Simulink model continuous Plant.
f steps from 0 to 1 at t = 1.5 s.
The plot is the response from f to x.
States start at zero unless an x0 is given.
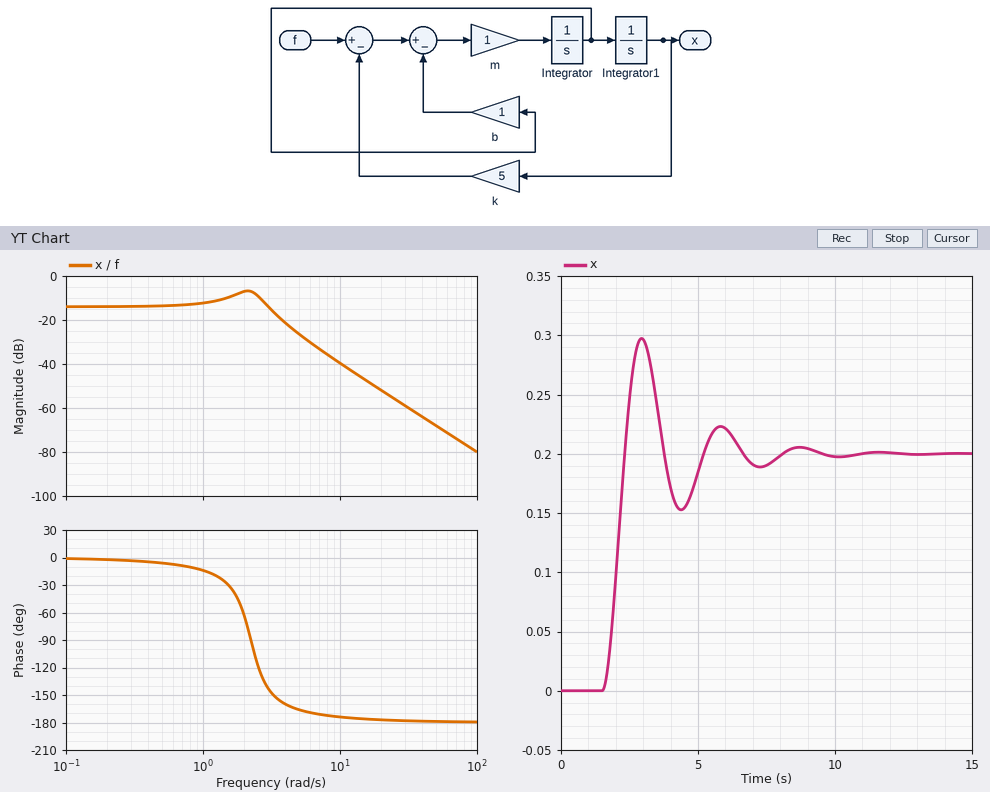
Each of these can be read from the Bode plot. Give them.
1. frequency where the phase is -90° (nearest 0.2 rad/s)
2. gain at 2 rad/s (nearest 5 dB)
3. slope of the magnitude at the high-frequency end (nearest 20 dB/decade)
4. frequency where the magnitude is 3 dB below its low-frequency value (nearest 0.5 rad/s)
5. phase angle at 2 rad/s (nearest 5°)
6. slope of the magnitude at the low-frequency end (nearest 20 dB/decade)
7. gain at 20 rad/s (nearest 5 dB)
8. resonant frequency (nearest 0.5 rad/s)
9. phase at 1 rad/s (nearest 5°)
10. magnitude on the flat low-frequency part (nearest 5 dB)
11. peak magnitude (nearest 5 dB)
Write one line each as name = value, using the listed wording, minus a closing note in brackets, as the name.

frequency where the phase is -90° = 2.2 rad/s
gain at 2 rad/s = -5 dB
slope of the magnitude at the high-frequency end = -40 dB/decade
frequency where the magnitude is 3 dB below its low-frequency value = 3.5 rad/s
phase angle at 2 rad/s = -65°
slope of the magnitude at the low-frequency end = 0 dB/decade
gain at 20 rad/s = -50 dB
resonant frequency = 2.0 rad/s
phase at 1 rad/s = -15°
magnitude on the flat low-frequency part = -15 dB
peak magnitude = -5 dB
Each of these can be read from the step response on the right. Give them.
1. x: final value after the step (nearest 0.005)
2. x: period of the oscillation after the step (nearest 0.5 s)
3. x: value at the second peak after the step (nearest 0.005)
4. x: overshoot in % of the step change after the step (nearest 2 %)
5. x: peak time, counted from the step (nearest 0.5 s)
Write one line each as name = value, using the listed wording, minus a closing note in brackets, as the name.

x: final value after the step = 0.200
x: period of the oscillation after the step = 3.0 s
x: value at the second peak after the step = 0.225
x: overshoot in % of the step change after the step = 48 %
x: peak time, counted from the step = 1.5 s
